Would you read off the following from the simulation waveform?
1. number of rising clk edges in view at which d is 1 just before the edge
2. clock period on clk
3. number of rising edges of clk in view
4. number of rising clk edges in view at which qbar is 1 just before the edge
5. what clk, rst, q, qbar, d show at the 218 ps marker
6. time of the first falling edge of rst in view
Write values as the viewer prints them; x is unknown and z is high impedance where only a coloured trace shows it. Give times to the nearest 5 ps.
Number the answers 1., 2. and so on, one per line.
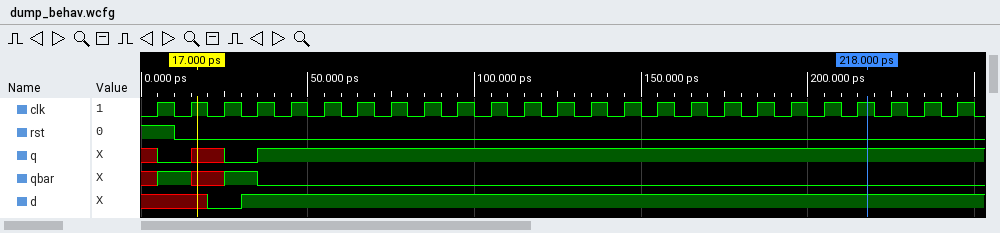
1. 22
2. 10 ps
3. 25
4. 2
5. clk=1, rst=0, q=1, qbar=0, d=1
6. 10 ps
